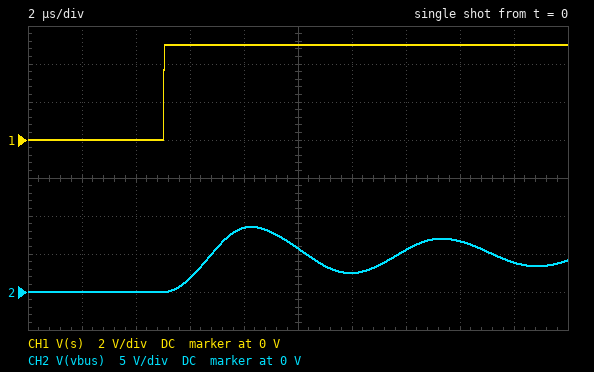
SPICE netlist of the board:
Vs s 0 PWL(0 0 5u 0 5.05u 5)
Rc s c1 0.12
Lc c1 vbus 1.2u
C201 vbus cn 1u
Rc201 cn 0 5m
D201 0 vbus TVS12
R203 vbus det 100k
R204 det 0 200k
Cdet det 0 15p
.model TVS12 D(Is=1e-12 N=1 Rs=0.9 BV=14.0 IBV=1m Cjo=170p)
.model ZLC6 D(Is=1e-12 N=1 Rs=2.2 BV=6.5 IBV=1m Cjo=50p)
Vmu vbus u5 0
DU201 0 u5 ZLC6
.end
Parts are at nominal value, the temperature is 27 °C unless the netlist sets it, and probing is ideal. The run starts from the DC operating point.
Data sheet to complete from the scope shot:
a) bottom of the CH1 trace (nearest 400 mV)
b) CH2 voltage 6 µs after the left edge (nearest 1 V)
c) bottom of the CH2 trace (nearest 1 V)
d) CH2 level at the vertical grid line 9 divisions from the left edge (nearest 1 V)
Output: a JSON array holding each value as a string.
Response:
["0 V", "2 V", "0 V", "4 V"]
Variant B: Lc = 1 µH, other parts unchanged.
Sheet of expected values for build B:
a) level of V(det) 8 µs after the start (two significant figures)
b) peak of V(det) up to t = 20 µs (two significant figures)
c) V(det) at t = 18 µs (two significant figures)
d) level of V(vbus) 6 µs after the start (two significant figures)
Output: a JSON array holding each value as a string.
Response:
["4.2 V", "4.9 V", "2.7 V", "2.1 V"]
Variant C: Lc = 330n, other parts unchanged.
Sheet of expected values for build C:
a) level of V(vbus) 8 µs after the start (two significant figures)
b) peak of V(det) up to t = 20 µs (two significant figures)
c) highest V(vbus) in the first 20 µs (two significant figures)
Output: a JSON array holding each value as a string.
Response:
["4.2 V", "4.1 V", "8.3 V"]
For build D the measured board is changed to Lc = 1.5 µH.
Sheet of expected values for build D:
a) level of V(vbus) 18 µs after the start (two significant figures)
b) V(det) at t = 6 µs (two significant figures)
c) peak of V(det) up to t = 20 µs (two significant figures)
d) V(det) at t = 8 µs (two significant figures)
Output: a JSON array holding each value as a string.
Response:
["5.9 V", "260 mV", "5.1 V", "3.5 V"]
